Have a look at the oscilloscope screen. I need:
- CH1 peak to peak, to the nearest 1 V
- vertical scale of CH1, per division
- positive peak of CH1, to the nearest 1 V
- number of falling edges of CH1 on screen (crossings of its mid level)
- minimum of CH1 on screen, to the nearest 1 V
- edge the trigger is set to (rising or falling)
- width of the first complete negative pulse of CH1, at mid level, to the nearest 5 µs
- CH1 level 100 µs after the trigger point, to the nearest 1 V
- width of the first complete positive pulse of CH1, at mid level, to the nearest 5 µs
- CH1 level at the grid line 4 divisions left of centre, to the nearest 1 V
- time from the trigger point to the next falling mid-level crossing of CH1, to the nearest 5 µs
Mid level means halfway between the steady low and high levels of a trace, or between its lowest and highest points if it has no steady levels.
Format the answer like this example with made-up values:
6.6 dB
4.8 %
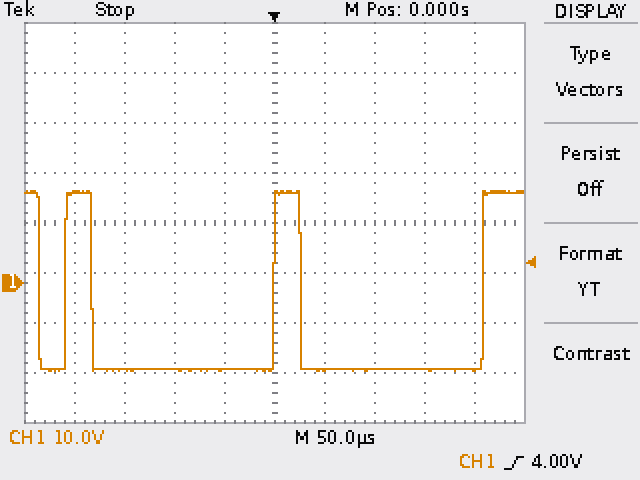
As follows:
36 V
10 V
18 V
3
-18 V
rising
25 µs
-17 V
25 µs
18 V
25 µs
